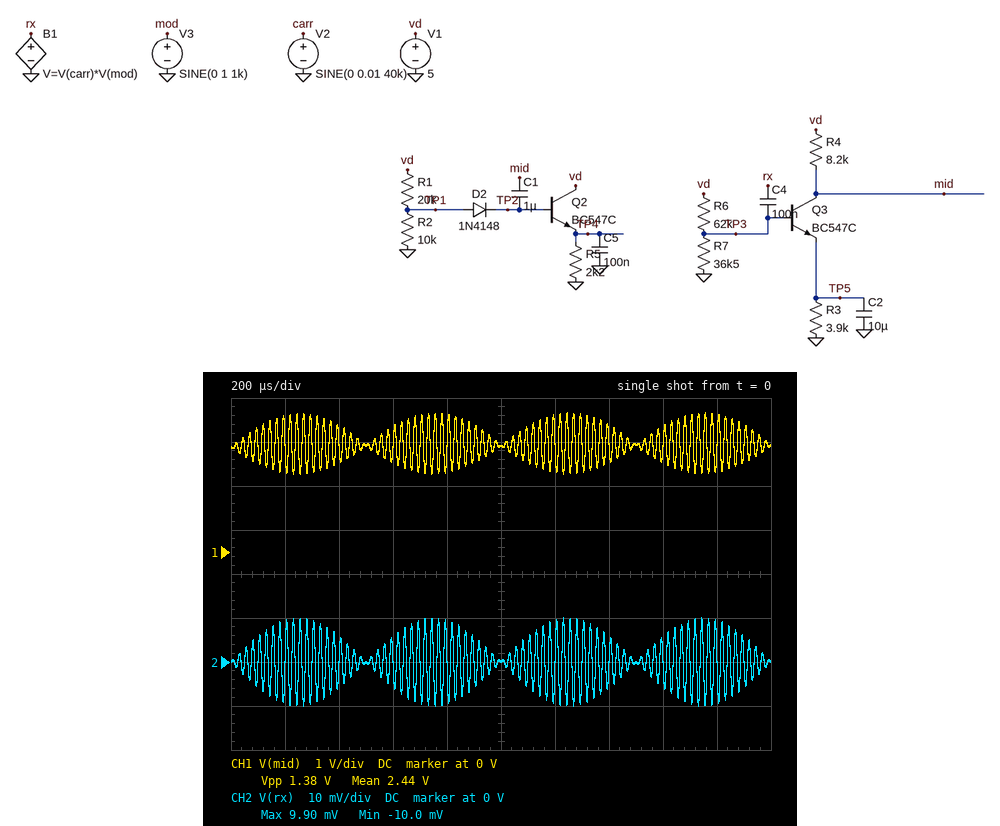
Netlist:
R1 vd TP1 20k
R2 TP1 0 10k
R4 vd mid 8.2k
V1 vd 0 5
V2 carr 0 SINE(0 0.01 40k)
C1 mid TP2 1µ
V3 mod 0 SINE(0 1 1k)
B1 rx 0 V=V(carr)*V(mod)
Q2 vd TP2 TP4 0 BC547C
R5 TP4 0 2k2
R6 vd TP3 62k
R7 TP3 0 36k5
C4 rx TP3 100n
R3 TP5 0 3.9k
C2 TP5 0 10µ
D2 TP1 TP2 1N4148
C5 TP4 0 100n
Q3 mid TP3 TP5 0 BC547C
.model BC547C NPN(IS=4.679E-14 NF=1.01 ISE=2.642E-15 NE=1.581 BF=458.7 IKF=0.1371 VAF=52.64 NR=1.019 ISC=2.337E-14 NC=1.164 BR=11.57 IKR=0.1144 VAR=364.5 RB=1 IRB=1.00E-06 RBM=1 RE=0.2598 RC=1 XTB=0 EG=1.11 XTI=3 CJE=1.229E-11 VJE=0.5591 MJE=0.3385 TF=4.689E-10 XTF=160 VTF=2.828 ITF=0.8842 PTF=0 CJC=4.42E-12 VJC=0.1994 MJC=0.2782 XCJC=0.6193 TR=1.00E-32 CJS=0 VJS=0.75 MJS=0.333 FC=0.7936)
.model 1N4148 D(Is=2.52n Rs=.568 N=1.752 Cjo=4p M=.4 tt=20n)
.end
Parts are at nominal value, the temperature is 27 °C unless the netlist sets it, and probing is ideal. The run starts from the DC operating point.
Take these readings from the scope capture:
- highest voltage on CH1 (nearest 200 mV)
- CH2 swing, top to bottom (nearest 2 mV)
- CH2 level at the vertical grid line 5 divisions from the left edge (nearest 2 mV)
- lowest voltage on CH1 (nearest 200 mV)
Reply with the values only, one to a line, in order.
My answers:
3.2 V
20 mV
0 V
1.8 V
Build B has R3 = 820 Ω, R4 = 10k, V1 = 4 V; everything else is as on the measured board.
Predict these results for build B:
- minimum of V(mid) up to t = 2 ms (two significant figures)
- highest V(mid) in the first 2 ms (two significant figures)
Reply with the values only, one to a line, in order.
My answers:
330 mV
390 mV
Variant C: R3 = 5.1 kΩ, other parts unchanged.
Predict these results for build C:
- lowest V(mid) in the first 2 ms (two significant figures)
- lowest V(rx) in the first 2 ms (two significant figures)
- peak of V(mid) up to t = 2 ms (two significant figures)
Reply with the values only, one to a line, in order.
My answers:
2.5 V
-10 mV
3.6 V
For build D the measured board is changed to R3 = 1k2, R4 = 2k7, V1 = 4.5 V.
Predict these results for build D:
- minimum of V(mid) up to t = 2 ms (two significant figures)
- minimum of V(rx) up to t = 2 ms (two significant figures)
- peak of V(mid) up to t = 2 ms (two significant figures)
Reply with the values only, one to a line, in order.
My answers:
1.5 V
-10 mV
2.9 V
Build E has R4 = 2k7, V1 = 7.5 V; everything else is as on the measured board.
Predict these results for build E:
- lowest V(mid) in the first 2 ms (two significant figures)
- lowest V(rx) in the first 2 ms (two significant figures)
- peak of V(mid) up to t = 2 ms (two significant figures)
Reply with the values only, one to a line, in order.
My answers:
5.5 V
-10 mV
6.5 V
